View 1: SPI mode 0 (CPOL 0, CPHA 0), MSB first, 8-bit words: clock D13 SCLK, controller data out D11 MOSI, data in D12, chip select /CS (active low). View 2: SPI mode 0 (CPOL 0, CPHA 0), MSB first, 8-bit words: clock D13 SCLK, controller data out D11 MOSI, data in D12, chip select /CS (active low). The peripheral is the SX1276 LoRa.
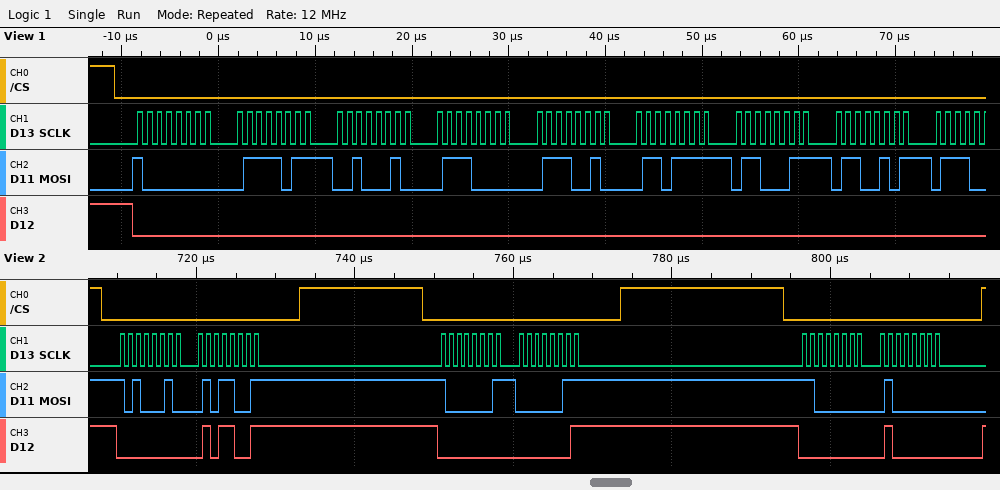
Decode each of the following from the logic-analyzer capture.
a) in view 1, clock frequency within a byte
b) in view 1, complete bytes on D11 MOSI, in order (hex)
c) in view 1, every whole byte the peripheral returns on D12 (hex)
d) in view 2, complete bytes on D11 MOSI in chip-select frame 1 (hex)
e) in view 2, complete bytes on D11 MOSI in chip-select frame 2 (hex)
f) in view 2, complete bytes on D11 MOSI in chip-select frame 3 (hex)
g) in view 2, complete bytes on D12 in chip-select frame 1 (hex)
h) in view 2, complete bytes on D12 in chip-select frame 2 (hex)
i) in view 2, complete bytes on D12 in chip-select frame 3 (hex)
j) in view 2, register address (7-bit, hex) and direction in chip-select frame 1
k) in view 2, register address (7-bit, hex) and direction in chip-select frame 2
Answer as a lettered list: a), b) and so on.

a) 1 MHz
b) 0x80 0x7B 0x22 0x70 0x72 0x6F 0x63 0x65
c) 0x00 0x00 0x00 0x00 0x00 0x00 0x00 0x00
d) A2 59
e) 81 03
f) C0 40
g) 00 59
h) 00 01
i) 00 40
j) 0x22 write
k) 0x01 write
